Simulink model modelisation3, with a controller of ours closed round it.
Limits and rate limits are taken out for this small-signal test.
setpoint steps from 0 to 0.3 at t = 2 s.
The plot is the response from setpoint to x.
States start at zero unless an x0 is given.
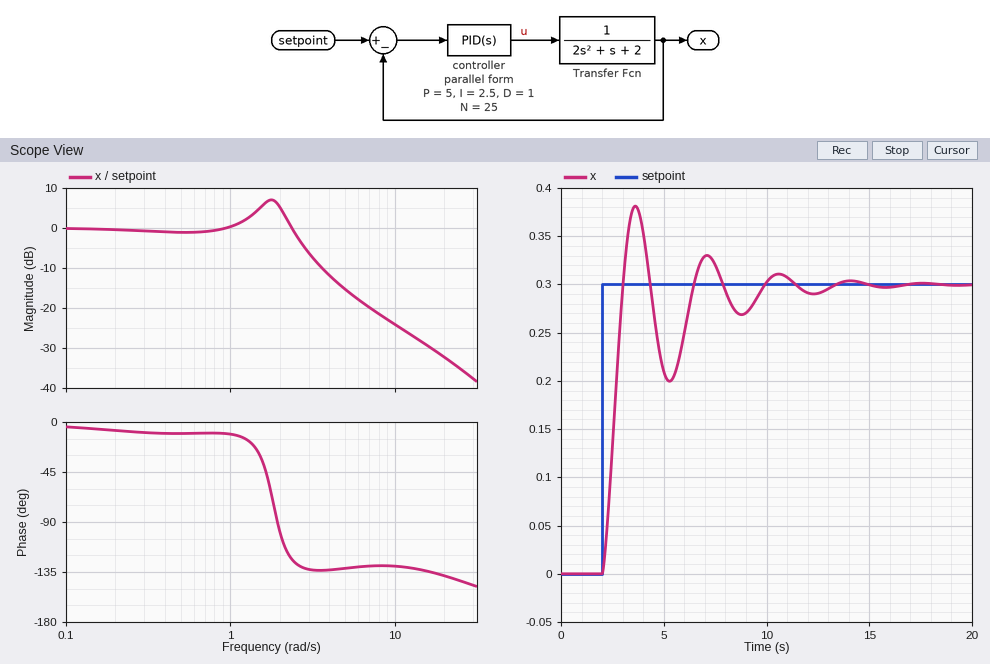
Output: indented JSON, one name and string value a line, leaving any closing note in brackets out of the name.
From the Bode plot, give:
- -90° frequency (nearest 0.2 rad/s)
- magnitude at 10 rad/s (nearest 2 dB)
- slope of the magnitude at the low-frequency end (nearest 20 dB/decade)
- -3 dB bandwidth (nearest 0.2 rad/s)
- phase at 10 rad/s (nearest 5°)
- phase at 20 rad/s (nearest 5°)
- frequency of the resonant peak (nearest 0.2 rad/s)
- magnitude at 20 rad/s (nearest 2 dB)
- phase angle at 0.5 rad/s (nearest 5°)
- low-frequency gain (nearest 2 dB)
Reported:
{
  "-90° frequency": "2.0 rad/s",
  "magnitude at 10 rad/s": "-24 dB",
  "slope of the magnitude at the low-frequency end": "0 dB/decade",
  "-3 dB bandwidth": "2.6 rad/s",
  "phase at 10 rad/s": "-130°",
  "phase at 20 rad/s": "-140°",
  "frequency of the resonant peak": "1.8 rad/s",
  "magnitude at 20 rad/s": "-32 dB",
  "phase angle at 0.5 rad/s": "-10°",
  "low-frequency gain": "0 dB"
}
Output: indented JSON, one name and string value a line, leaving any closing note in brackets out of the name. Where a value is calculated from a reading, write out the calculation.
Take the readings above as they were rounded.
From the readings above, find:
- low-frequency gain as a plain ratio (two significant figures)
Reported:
{
  "low-frequency gain as a plain ratio": "10^(0 / 20) = 1.0"
}
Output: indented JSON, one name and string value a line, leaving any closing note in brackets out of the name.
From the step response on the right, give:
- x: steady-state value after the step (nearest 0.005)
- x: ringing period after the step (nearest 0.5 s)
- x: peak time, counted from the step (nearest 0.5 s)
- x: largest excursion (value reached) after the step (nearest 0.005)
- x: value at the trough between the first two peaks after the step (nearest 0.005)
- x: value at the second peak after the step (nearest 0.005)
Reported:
{
  "x: steady-state value after the step": "0.300",
  "x: ringing period after the step": "3.5 s",
  "x: peak time, counted from the step": "1.5 s",
  "x: largest excursion (value reached) after the step": "0.380",
  "x: value at the trough between the first two peaks after the step": "0.200",
  "x: value at the second peak after the step": "0.330"
}
